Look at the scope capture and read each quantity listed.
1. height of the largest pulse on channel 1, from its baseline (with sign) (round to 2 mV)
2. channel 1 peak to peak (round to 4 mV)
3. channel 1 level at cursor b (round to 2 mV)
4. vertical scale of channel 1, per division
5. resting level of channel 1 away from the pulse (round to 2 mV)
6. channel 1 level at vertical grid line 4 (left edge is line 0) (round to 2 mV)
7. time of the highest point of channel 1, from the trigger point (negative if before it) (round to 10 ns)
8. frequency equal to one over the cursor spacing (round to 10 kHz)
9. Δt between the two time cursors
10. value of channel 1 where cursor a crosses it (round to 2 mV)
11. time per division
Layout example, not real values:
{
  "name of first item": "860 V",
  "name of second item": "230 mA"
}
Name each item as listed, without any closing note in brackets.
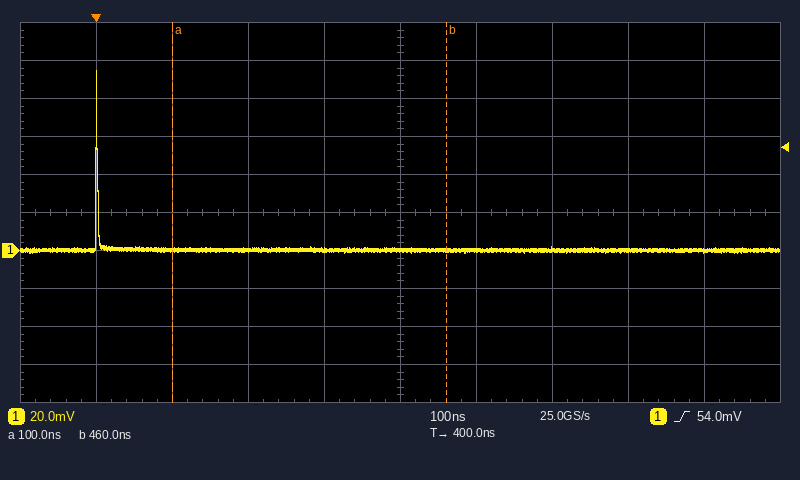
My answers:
{
  "height of the largest pulse on channel 1, from its baseline (with sign)": "+94 mV",
  "channel 1 peak to peak": "96 mV",
  "channel 1 level at cursor b": "0 mV",
  "vertical scale of channel 1, per division": "20 mV",
  "resting level of channel 1 away from the pulse": "0 mV",
  "channel 1 level at vertical grid line 4 (left edge is line 0)": "0 mV",
  "time of the highest point of channel 1, from the trigger point (negative if before it)": "0 ns",
  "frequency equal to one over the cursor spacing": "2.78 MHz",
  "Δt between the two time cursors": "360 ns",
  "value of channel 1 where cursor a crosses it": "0 mV",
  "time per division": "100 ns"
}
